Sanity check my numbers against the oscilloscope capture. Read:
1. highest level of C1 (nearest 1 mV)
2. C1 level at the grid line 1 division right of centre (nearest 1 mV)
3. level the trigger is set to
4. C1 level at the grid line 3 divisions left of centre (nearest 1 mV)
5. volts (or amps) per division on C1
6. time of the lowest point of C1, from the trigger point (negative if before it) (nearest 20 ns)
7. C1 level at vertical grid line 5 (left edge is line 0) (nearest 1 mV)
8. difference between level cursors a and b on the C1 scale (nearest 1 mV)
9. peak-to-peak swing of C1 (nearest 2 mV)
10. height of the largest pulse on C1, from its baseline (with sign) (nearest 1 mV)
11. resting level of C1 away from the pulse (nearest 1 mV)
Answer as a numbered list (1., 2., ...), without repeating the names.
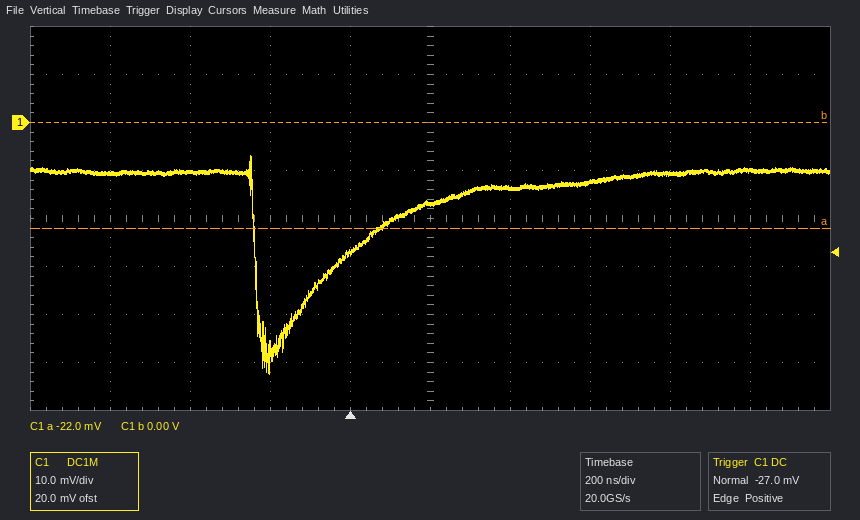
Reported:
1. -7 mV
2. -14 mV
3. -27.0 mV
4. -10 mV
5. 10 mV
6. -200 ns
7. -17 mV
8. 22 mV
9. 46 mV
10. -42 mV
11. -10 mV
